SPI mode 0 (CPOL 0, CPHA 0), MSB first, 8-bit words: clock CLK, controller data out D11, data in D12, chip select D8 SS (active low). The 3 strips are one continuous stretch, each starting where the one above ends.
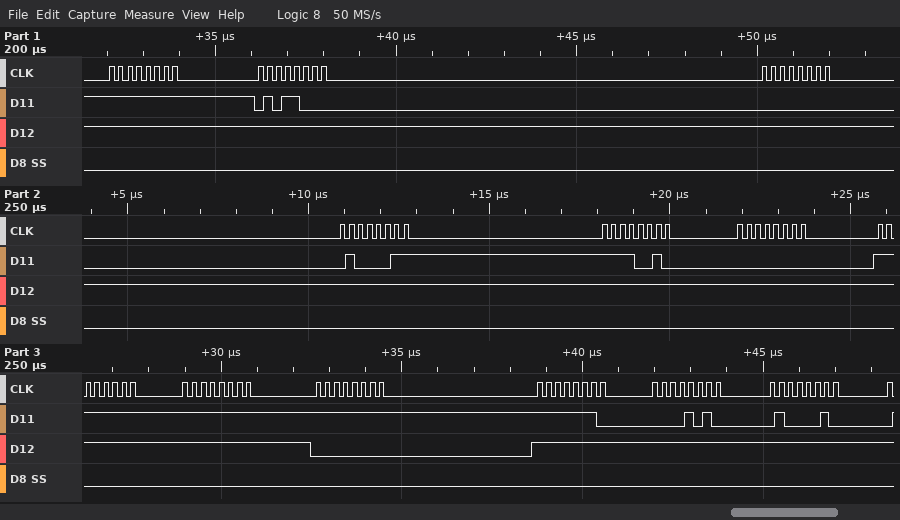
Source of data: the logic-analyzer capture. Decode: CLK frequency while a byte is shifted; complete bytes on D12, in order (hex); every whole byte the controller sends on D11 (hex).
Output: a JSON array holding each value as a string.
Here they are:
["4 MHz", "FF FF FF FF FF FF FF FF 00 FF FF FF", "FF 58 00 43 F2 00 FF FF FF FE 0A 42"]
